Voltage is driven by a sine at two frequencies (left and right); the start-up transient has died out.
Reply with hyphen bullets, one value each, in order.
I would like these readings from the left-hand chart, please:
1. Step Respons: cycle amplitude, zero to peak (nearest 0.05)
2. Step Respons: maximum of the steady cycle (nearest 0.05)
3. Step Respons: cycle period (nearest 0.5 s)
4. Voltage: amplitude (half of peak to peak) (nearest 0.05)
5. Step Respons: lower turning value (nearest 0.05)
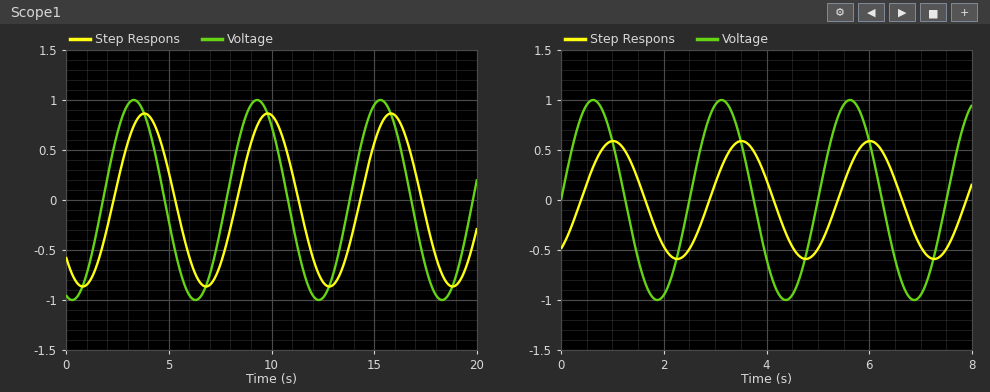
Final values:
- 0.85
- 0.85
- 6.0 s
- 1.00
- -0.85
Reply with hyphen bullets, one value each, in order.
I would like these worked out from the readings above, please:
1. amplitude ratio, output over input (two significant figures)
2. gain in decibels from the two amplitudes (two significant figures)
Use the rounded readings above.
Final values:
- 0.85
- -1.4 dB
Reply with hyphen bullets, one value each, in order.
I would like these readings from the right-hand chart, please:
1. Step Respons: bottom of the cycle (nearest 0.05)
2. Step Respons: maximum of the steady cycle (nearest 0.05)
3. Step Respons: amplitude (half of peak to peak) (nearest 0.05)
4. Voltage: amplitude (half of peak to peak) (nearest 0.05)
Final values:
- -0.60
- 0.60
- 0.60
- 1.00
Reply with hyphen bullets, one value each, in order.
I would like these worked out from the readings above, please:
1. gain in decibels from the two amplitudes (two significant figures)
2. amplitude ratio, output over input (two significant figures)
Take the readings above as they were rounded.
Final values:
- -4.4 dB
- 0.60
